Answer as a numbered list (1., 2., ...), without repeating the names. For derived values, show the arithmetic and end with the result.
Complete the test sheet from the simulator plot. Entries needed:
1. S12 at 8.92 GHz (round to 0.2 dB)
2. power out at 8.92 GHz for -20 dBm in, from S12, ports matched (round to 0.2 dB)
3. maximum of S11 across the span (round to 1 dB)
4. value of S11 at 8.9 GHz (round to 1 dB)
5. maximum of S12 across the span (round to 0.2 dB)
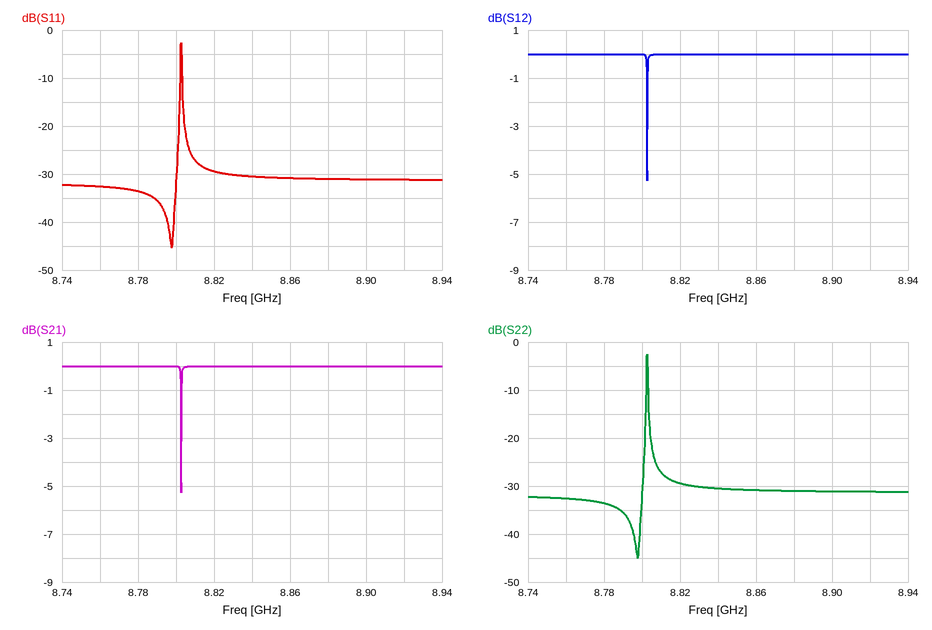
1. 0.0 dB
2. -20 dBm + (0.0 dB) = -20.0 dBm
3. -3 dB
4. -31 dB
5. 0.0 dB
